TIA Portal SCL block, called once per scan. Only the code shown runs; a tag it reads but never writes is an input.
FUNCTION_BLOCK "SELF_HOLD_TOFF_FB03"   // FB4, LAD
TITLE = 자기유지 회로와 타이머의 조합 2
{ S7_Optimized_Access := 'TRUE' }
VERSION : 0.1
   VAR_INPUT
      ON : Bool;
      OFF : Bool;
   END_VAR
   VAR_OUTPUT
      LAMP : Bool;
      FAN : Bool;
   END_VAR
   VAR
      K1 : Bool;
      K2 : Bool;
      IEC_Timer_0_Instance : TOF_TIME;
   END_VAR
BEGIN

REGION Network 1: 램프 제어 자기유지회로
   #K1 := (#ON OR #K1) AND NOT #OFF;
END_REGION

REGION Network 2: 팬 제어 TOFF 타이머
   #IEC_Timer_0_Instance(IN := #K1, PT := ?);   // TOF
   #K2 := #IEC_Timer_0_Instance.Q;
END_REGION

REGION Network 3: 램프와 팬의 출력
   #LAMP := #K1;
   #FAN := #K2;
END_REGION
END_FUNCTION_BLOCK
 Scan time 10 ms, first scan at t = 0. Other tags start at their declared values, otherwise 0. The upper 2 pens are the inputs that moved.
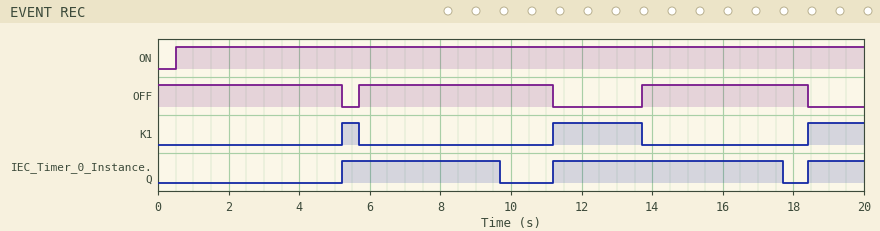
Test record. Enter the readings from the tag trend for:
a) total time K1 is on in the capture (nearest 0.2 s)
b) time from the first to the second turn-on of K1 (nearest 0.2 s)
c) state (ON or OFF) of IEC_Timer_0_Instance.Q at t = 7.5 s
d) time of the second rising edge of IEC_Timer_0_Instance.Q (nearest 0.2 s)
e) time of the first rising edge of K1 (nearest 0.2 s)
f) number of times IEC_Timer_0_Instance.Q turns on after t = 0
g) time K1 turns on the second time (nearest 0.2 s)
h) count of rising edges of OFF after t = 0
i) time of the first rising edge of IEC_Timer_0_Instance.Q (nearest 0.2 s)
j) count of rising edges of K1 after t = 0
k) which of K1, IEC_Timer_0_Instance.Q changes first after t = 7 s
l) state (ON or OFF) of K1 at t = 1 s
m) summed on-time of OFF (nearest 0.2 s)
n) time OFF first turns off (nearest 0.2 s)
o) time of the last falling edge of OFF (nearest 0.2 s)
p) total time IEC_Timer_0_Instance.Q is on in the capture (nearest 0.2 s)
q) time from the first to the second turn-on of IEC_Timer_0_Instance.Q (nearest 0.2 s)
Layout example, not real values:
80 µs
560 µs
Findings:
4.6 s
6.0 s
ON
11.2 s
5.2 s
3
11.2 s
2
5.2 s
3
IEC_Timer_0_Instance.Q
OFF
15.4 s
5.2 s
18.4 s
12.6 s
6.0 s
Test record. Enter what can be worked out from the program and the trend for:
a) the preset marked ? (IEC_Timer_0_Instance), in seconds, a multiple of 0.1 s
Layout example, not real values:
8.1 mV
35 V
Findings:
4.0 s
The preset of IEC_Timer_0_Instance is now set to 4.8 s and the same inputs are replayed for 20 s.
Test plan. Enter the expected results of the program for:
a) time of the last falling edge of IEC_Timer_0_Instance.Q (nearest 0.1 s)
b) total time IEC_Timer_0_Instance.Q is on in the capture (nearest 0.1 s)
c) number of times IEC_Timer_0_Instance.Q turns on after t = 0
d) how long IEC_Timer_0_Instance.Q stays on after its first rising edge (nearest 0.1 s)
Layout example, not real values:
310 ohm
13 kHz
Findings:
10.5 s
14.1 s
2
5.3 s
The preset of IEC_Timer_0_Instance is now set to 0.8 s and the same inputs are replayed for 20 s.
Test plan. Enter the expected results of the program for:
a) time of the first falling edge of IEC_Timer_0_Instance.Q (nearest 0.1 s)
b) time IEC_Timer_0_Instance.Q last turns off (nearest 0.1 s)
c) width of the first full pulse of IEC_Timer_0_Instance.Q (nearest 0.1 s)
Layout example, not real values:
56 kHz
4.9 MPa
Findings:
6.5 s
14.5 s
1.3 s
